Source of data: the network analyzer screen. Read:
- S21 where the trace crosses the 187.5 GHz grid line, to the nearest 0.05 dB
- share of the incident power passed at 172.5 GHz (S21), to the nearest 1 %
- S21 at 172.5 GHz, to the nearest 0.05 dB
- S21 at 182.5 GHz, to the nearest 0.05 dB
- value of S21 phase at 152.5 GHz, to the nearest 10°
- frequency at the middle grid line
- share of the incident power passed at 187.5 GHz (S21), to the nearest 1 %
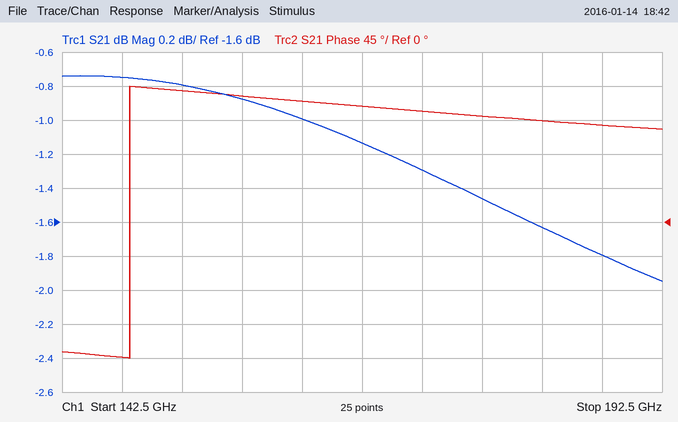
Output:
-1.80 dB
74 %
-1.30 dB
-1.65 dB
170°
167.5 GHz
66 %
